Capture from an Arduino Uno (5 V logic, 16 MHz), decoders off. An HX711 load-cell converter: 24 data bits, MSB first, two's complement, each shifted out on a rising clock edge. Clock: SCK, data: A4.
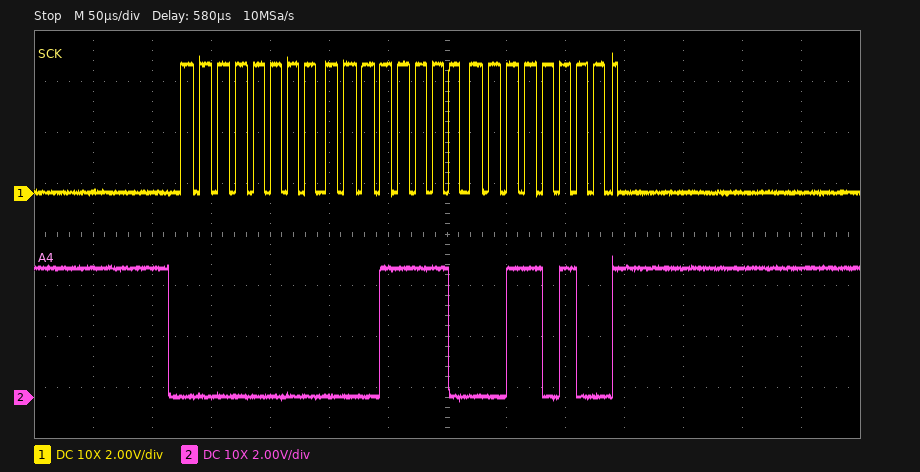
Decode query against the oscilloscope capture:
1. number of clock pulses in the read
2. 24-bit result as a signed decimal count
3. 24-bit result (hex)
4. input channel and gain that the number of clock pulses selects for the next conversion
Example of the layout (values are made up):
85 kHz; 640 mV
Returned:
25; 7732; 0x001E34; channel A, gain 128
